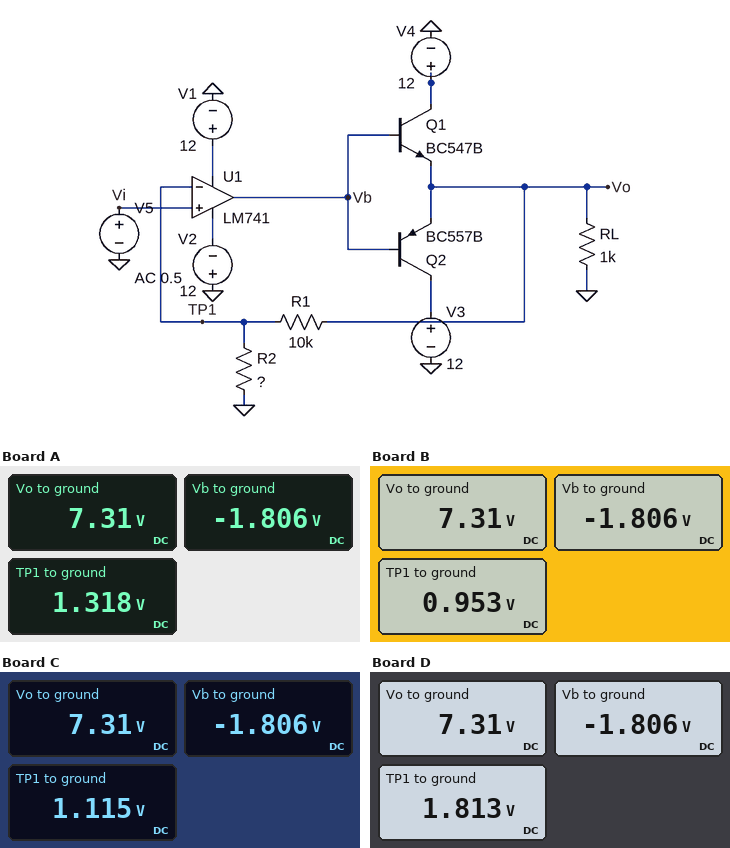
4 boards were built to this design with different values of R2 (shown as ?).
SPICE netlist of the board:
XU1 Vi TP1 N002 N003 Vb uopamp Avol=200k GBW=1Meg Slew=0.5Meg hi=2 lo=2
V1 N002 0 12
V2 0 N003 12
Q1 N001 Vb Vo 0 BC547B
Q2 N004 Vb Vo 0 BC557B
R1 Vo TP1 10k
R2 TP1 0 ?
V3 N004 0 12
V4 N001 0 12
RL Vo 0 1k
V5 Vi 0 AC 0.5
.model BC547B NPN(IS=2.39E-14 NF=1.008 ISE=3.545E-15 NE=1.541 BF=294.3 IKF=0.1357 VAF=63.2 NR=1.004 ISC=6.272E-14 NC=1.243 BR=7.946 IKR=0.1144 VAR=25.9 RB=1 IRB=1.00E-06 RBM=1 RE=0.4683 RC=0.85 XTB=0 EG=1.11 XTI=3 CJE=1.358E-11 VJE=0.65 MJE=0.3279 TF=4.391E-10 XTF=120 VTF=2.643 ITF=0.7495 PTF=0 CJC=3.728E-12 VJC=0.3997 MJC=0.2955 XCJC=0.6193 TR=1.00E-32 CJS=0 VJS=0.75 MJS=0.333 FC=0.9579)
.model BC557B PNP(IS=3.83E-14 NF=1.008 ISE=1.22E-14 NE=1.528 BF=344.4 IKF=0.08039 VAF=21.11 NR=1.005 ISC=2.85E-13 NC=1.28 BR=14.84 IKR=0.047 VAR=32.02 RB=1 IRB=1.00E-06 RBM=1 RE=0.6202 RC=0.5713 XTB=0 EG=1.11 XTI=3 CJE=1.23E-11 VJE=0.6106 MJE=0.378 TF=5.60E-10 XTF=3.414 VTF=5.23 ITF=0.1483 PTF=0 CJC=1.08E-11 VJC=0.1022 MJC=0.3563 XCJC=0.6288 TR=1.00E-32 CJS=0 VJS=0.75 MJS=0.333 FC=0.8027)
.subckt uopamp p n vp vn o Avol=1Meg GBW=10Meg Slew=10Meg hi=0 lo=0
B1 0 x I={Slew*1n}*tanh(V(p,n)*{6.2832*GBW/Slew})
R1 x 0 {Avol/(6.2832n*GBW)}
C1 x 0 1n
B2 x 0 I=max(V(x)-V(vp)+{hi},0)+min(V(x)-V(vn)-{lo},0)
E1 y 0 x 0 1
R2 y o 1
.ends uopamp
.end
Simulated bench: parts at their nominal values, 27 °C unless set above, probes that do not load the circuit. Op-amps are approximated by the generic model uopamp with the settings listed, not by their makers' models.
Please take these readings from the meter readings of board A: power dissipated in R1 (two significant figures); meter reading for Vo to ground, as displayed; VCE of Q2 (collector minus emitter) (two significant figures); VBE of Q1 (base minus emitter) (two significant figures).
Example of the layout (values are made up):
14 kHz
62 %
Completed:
3.6 mW
7.31 V
4.7 V
-9.1 V
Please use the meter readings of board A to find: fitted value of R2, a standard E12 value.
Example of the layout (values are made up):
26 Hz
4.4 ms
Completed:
2.2 kΩ
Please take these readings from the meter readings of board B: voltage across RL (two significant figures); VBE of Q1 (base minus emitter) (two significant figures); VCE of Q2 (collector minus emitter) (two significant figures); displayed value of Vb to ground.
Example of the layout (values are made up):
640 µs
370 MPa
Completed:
7.3 V
-9.1 V
4.7 V
-1.806 V
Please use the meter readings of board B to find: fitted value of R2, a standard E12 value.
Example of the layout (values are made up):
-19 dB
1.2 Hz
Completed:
1.5 kΩ
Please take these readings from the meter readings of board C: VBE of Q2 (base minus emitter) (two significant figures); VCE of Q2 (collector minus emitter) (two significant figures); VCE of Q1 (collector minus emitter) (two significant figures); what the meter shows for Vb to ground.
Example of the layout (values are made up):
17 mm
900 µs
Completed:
-9.1 V
4.7 V
4.7 V
-1.806 V
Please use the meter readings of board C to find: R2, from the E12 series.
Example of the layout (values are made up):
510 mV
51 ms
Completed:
1.8 kΩ
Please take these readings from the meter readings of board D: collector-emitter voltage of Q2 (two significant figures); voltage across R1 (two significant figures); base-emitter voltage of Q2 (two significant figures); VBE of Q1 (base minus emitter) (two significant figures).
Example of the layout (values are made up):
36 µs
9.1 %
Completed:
4.7 V
5.5 V
-9.1 V
-9.1 V
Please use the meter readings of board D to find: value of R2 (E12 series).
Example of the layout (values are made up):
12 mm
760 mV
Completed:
3.3 kΩ
